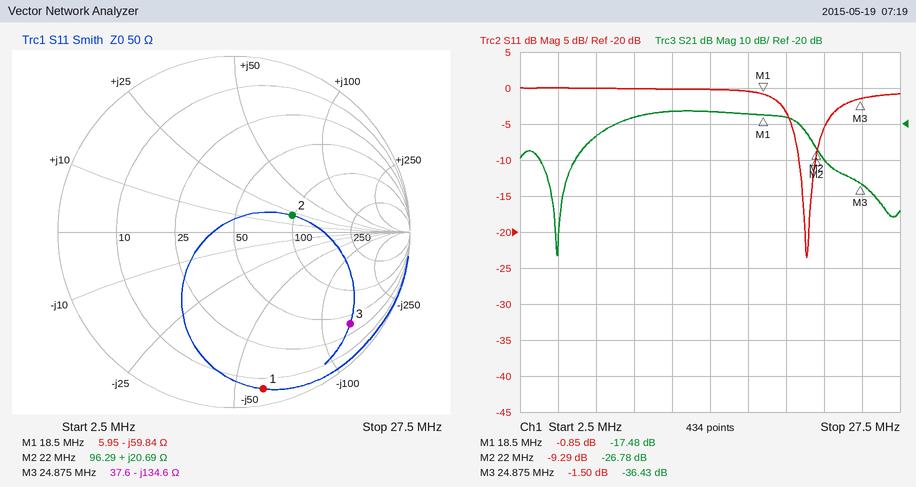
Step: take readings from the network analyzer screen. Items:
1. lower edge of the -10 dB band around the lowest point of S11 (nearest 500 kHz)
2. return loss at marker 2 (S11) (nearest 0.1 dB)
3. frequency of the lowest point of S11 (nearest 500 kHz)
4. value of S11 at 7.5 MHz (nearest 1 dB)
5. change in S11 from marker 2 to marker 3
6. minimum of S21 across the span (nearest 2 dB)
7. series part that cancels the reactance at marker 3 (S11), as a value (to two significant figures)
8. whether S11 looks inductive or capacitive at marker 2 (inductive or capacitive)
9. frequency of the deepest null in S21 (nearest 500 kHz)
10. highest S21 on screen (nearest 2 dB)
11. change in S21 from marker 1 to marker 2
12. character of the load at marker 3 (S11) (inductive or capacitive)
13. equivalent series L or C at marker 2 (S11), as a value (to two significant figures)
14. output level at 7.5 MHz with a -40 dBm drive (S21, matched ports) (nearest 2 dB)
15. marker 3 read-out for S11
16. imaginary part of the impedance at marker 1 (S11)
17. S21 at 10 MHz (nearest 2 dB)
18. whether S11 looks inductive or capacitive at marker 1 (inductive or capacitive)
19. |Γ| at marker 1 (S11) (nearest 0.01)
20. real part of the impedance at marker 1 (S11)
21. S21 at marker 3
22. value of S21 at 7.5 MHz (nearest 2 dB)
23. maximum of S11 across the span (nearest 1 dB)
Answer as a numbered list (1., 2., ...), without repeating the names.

1. 21.0 MHz
2. 9.3 dB
3. 21.5 MHz
4. 0 dB
5. 7.79 dB
6. -56 dB
7. 860 nH
8. inductive
9. 5.0 MHz
10. -16 dB
11. -9.30 dB
12. capacitive
13. 150 nH
14. -64 dBm
15. -1.50 dB
16. -59.84 Ω
17. -18 dB
18. capacitive
19. 0.91
20. 5.95 Ω
21. -36.43 dB
22. -24 dB
23. 0 dB
